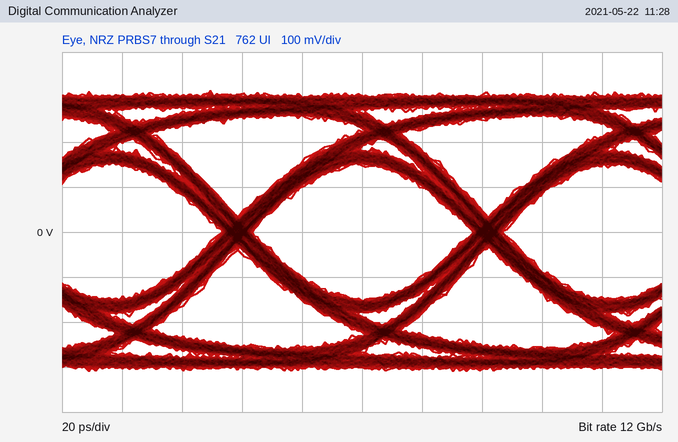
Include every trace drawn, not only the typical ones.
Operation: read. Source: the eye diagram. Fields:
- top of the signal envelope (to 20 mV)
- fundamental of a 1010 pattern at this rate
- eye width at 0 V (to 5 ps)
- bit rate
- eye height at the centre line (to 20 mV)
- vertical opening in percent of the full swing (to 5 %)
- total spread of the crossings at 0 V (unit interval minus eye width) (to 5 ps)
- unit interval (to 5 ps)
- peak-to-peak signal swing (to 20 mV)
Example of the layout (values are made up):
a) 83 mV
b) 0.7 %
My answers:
a) 320 mV
b) 6 GHz
c) 75 ps
d) 12 Gb/s
e) 300 mV
f) 50 %
g) 10 ps
h) 85 ps
i) 620 mV
